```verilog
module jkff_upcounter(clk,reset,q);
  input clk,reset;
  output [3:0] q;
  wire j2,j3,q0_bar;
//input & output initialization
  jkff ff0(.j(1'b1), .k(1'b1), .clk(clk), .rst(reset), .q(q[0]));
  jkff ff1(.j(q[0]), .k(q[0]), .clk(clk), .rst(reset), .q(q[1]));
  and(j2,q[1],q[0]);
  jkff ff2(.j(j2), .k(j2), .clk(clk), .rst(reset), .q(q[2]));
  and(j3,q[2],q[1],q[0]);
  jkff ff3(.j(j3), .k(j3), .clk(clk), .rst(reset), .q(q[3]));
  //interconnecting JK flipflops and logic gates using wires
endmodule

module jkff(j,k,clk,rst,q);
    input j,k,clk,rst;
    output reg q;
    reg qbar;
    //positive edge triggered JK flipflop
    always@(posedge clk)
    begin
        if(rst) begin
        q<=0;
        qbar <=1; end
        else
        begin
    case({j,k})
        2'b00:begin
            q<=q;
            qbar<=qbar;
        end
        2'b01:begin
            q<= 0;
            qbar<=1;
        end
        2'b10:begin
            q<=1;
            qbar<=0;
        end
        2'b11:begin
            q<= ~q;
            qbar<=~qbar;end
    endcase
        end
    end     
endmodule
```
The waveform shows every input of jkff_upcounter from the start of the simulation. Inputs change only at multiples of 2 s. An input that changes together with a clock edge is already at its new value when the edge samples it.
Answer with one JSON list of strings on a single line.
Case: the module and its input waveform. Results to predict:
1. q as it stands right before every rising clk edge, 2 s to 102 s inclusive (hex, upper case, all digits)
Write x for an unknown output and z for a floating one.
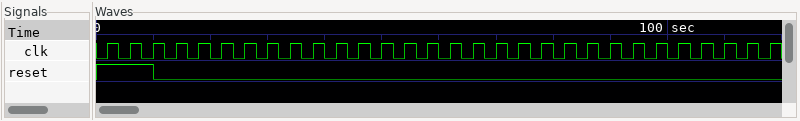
["x, 0, 0, 1, 2, 3, 4, 5, 6, 7, 8, 9, A, B, C, D, E, F, 0, 1, 2, 3, 4, 5, 6, 7"]
